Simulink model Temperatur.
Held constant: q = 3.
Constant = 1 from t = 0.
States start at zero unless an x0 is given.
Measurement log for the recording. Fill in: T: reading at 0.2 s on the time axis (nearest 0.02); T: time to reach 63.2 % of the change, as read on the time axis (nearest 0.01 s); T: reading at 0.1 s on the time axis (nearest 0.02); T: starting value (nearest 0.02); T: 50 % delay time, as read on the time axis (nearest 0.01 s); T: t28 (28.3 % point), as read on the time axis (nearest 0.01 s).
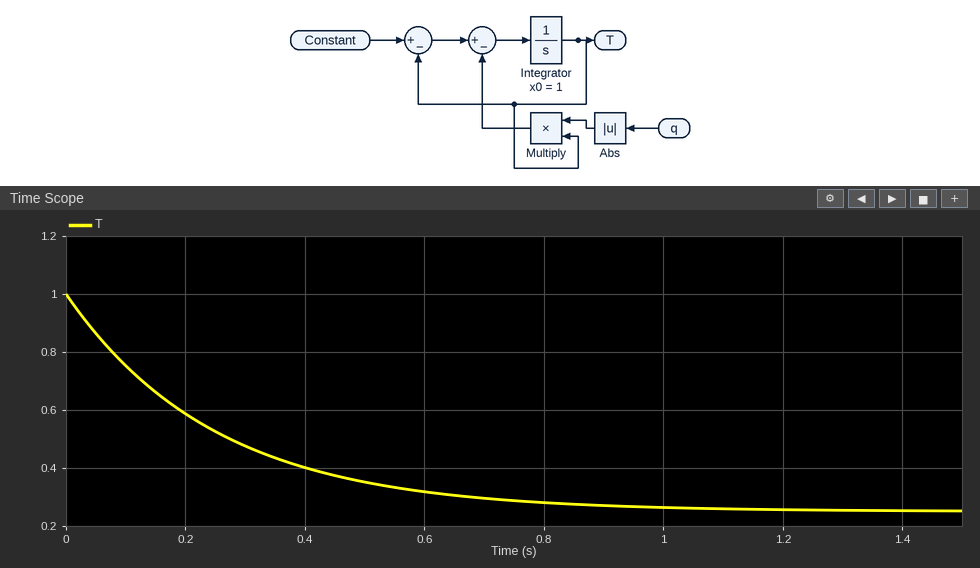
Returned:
0.58
0.25 s
0.76
1.00
0.17 s
0.08 s
